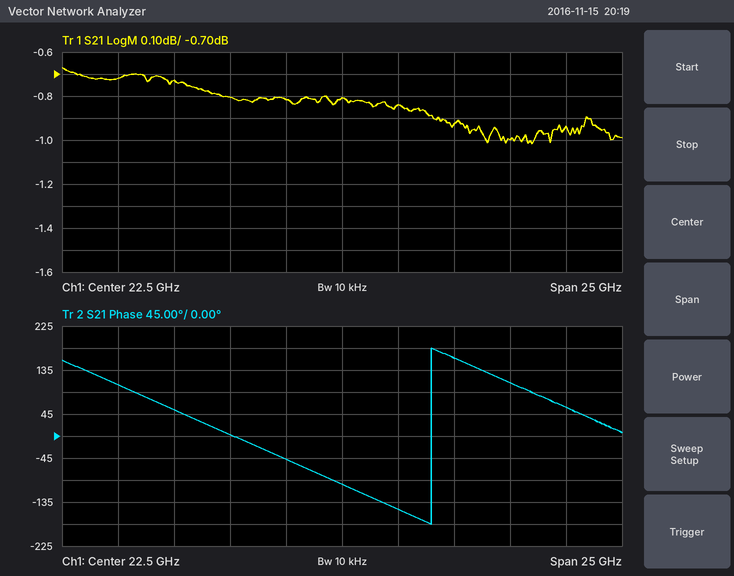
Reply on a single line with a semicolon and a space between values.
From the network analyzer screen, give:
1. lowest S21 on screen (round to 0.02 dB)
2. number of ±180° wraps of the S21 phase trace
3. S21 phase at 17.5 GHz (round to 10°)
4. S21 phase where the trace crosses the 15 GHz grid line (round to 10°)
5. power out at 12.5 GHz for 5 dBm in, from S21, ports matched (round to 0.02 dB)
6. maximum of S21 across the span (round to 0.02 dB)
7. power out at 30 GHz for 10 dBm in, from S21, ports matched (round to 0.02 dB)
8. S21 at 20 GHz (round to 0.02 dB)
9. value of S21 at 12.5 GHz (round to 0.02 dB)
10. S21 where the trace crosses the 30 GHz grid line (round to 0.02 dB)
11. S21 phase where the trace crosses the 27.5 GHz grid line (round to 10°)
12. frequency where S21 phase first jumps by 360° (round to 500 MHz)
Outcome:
-1.02 dB; 1; 0°; 50°; 4.28 dBm; -0.68 dB; 9.00 dBm; -0.82 dB; -0.72 dB; -1.00 dB; 160°; 26.5 GHz
